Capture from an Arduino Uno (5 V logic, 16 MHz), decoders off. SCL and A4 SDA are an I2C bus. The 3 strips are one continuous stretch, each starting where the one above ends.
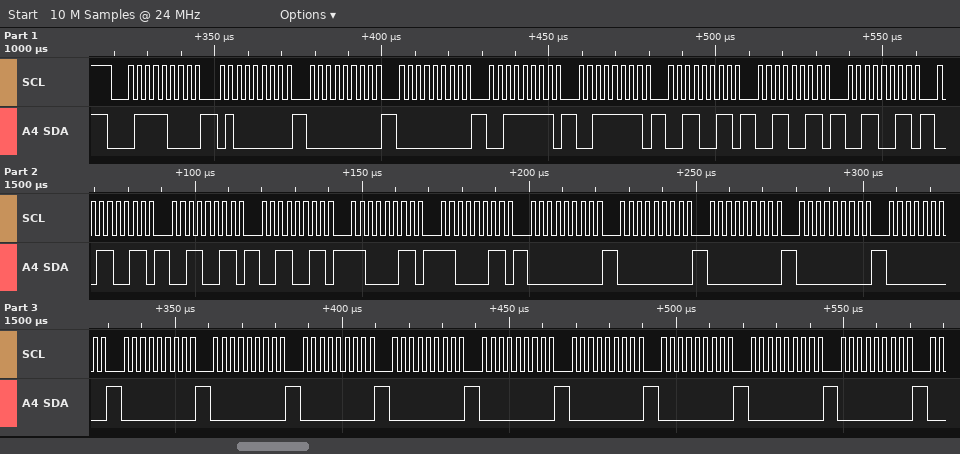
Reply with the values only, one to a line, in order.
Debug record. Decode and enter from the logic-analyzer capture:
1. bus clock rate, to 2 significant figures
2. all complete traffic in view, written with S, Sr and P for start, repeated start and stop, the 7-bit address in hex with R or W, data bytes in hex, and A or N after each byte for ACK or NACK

400 kHz
S 3CW A 40 A 00 A 00 A 3F A 3F A 33 A 33 A 33 A 33 A 33 A 33 A C3 A C3 A 00 A 00 A 00 A 00 A 00 A 00 A 00 A 00 A 00 A 00 A 00 A 00 A 00 A 00 A
